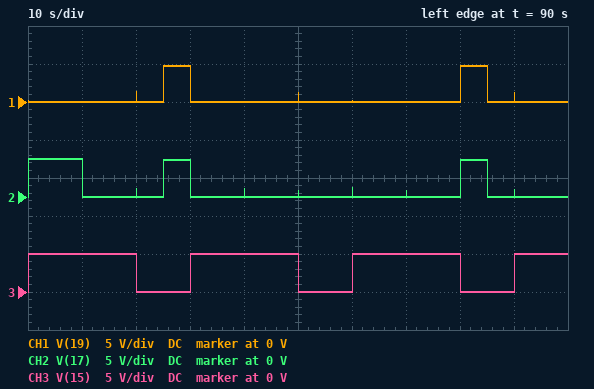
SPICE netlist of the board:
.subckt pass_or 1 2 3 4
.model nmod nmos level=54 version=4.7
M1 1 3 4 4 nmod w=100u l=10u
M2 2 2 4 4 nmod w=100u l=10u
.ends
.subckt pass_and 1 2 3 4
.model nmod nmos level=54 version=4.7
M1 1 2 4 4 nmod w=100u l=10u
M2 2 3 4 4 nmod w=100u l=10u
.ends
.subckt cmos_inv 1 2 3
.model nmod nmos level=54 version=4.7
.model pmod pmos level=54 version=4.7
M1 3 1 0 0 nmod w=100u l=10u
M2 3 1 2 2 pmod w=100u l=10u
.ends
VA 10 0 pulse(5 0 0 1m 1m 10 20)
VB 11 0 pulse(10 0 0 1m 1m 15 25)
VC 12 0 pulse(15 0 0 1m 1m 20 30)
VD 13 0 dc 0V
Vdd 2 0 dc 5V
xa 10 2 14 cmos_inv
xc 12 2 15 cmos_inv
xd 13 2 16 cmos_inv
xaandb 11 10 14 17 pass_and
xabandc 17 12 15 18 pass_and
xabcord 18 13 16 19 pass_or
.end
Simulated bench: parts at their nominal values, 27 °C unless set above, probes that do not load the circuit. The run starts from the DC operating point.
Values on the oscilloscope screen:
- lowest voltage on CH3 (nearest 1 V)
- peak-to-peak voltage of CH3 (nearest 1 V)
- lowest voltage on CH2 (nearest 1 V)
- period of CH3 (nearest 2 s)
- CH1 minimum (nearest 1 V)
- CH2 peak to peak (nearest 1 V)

0 V
5 V
0 V
30 s
0 V
5 V
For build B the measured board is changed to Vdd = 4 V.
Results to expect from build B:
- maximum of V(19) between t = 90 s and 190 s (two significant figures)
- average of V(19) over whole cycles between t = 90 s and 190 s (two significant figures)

3.8 V
350 mV
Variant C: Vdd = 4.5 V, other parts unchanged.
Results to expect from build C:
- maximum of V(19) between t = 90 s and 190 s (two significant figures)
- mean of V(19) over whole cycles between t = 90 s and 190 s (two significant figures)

4.3 V
390 mV
